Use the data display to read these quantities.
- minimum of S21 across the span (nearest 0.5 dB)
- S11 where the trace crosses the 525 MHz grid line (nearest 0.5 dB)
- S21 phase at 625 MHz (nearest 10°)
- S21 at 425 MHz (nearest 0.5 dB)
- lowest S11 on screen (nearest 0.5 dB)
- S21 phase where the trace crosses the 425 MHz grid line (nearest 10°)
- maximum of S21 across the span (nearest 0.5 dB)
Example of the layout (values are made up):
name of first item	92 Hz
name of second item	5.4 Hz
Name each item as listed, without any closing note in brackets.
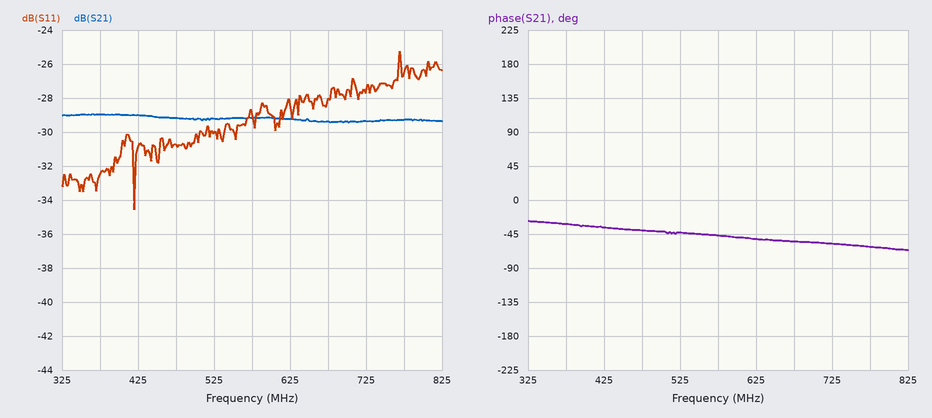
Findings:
minimum of S21 across the span	-29.5 dB
S11 where the trace crosses the 525 MHz grid line	-30.0 dB
S21 phase at 625 MHz	-50°
S21 at 425 MHz	-29.0 dB
lowest S11 on screen	-34.5 dB
S21 phase where the trace crosses the 425 MHz grid line	-40°
maximum of S21 across the span	-29.0 dB
